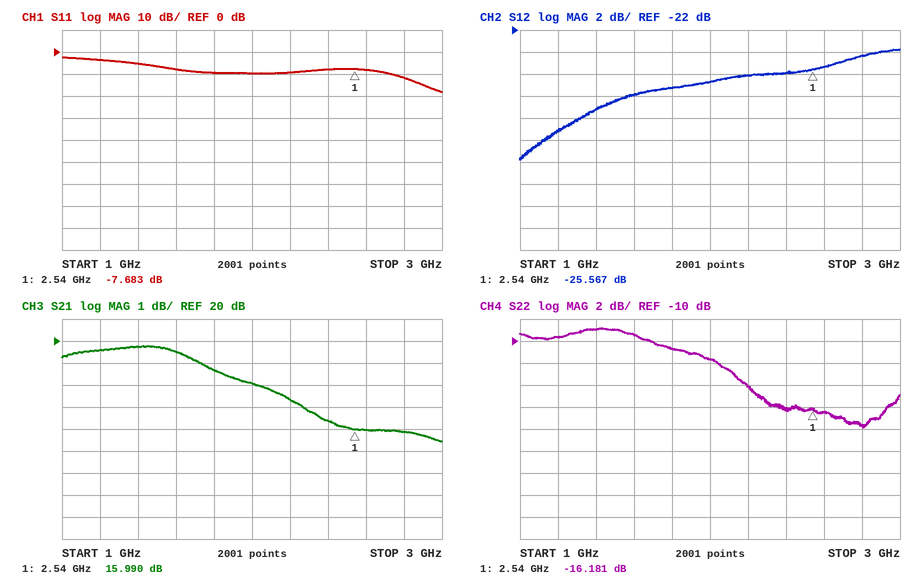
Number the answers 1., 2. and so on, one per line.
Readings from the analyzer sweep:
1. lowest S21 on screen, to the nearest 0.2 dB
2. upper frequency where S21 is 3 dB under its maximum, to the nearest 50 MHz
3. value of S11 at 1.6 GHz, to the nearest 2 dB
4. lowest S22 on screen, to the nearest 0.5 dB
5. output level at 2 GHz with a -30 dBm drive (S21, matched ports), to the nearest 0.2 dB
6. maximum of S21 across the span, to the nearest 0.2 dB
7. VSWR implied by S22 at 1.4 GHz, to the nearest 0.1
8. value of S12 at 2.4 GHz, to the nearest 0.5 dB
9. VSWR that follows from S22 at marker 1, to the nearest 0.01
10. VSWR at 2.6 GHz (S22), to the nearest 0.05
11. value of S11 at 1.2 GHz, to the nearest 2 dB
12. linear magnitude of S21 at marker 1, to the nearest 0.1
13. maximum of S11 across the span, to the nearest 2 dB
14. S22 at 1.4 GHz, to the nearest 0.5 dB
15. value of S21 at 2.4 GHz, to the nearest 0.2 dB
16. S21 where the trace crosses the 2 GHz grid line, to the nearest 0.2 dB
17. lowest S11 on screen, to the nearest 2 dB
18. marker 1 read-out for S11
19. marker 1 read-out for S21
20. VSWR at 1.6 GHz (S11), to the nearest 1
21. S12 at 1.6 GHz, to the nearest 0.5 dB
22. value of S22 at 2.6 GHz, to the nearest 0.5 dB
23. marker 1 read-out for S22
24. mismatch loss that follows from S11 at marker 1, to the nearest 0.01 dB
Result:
1. 15.4 dB
2. 2.30 GHz
3. -8 dB
4. -18.0 dB
5. -12.0 dBm
6. 19.8 dB
7. 2.1
8. -26.0 dB
9. 1.37
10. 1.35
11. -4 dB
12. 6.3
13. -2 dB
14. -9.0 dB
15. 16.4 dB
16. 18.0 dB
17. -18 dB
18. -7.683 dB
19. 15.990 dB
20. 2
21. -28.0 dB
22. -16.5 dB
23. -16.181 dB
24. 0.81 dB
